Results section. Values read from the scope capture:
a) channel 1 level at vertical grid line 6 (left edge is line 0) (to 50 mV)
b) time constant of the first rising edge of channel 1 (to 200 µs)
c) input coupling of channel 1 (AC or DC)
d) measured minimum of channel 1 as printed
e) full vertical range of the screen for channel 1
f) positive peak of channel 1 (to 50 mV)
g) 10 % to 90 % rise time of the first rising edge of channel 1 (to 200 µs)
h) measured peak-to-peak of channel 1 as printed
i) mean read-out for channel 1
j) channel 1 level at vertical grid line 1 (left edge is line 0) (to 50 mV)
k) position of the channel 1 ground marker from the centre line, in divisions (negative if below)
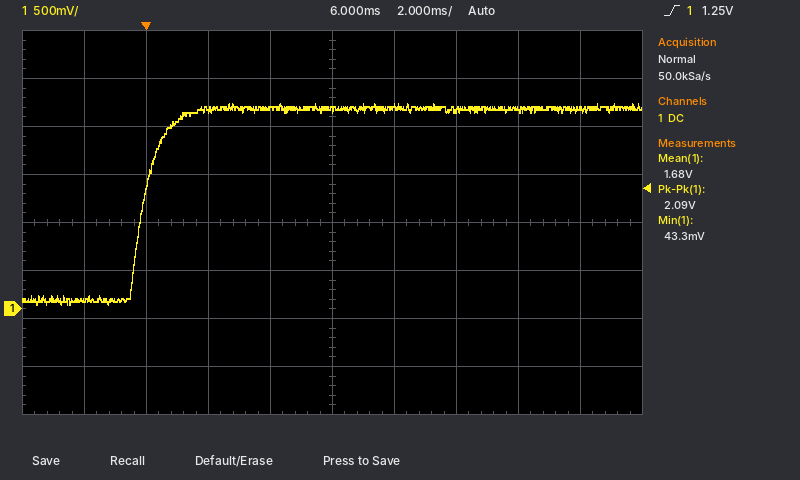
2.10 V
600 µs
DC
43.3 mV
4 V
2.15 V
1.2 ms
2.09 V
1.68 V
100 mV
-1.8 div
